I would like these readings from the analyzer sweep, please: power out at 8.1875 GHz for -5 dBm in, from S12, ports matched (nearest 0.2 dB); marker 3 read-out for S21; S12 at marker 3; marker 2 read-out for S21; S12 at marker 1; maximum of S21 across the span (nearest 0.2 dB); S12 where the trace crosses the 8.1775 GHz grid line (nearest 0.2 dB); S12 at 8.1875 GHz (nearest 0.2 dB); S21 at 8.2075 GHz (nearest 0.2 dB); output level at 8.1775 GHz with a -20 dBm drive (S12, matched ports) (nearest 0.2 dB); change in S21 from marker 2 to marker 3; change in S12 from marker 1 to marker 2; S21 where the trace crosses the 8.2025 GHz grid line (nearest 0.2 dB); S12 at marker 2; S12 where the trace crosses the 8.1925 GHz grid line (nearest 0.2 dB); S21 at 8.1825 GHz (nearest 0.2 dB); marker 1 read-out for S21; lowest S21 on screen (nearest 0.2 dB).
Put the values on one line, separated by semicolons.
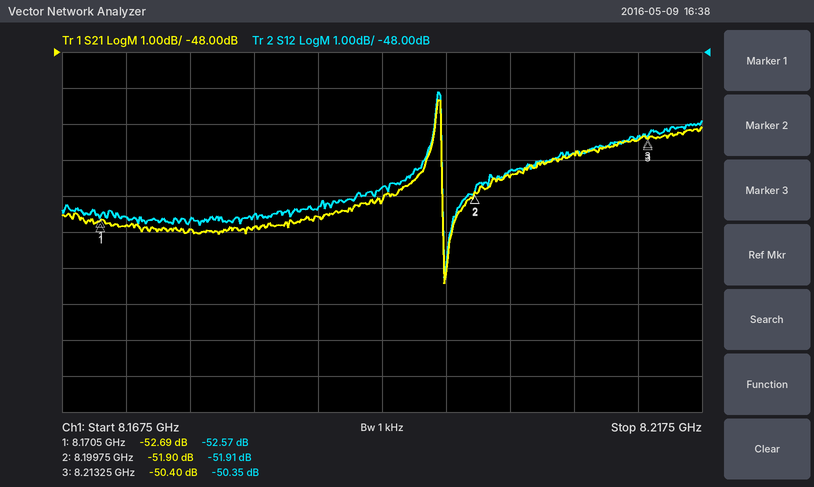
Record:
-57.4 dBm; -50.40 dB; -50.35 dB; -51.90 dB; -52.57 dB; -49.4 dB; -52.6 dB; -52.4 dB; -50.8 dB; -72.6 dBm; 1.50 dB; 0.66 dB; -51.4 dB; -51.91 dB; -51.8 dB; -52.8 dB; -52.69 dB; -54.4 dB
